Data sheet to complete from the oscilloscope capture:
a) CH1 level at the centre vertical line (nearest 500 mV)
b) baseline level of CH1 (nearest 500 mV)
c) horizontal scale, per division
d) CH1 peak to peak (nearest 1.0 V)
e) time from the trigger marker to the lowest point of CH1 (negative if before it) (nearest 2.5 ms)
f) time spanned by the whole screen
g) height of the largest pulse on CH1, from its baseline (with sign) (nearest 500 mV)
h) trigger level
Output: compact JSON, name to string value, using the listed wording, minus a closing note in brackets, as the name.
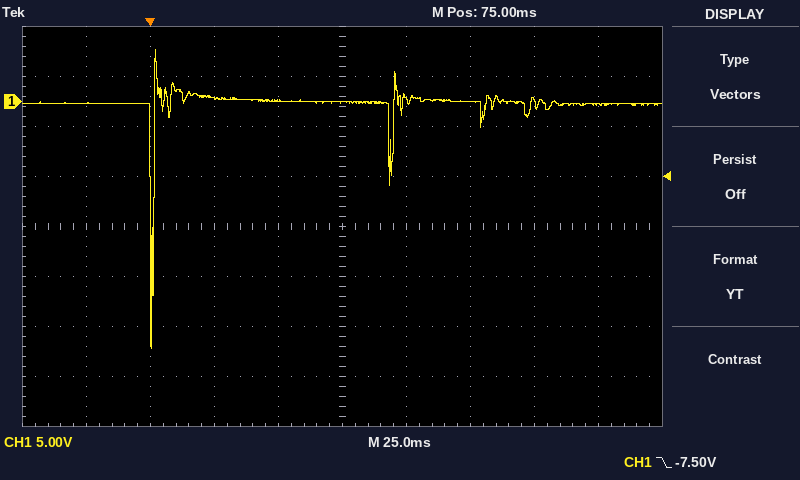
{"CH1 level at the centre vertical line": "0.0 V", "baseline level of CH1": "0.0 V", "horizontal scale, per division": "25 ms", "CH1 peak to peak": "30.0 V", "time from the trigger marker to the lowest point of CH1 (negative if before it)": "0.0 ms", "time spanned by the whole screen": "250 ms", "height of the largest pulse on CH1, from its baseline (with sign)": "-24.5 V", "trigger level": "-7.50 V"}
